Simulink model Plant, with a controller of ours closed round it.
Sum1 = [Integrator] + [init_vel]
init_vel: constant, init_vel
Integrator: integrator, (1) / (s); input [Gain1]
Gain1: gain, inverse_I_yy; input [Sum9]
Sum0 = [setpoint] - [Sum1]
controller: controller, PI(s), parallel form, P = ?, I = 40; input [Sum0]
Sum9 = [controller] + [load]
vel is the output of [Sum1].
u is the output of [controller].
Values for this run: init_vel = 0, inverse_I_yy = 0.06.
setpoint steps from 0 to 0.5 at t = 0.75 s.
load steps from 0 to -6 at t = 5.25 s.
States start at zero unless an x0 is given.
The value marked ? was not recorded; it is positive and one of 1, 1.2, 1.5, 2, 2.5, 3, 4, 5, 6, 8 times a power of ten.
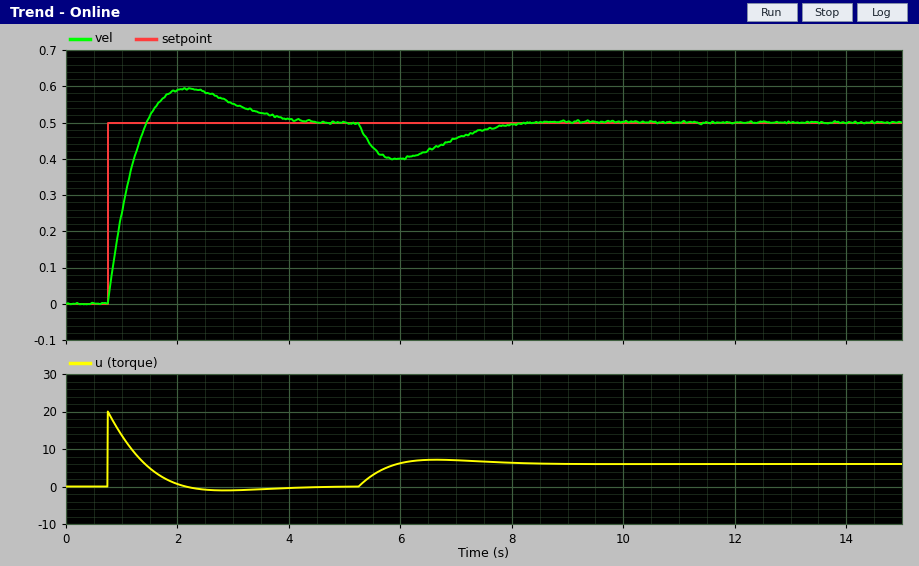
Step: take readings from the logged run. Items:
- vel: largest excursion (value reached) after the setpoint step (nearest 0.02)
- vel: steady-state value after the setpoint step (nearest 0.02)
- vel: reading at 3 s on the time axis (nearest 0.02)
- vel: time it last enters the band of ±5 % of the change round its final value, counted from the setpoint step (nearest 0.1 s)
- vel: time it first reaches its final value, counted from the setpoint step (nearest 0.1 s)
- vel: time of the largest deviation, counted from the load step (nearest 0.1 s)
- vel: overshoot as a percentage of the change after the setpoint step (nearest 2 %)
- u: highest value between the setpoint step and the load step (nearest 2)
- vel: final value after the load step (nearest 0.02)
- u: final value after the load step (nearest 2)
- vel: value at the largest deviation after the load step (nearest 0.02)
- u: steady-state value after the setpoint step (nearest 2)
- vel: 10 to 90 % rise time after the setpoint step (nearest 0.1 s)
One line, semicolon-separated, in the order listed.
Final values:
0.60; 0.50; 0.56; 2.8 s; 0.7 s; 0.7 s; 18 %; 20; 0.50; 6; 0.40; 0; 0.5 s
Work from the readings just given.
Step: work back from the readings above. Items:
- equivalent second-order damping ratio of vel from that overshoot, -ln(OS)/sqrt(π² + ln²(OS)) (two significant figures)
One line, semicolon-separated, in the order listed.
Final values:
0.48
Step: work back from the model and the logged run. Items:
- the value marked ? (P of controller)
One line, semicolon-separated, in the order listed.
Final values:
40
